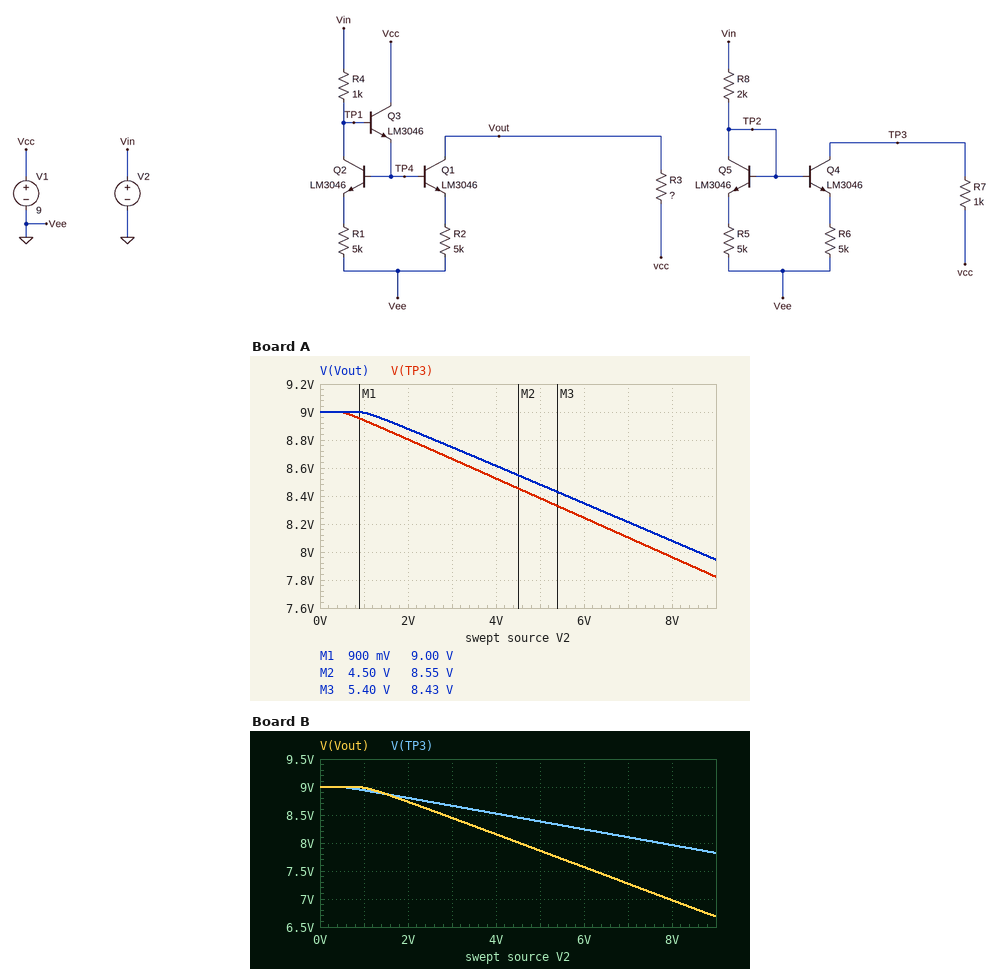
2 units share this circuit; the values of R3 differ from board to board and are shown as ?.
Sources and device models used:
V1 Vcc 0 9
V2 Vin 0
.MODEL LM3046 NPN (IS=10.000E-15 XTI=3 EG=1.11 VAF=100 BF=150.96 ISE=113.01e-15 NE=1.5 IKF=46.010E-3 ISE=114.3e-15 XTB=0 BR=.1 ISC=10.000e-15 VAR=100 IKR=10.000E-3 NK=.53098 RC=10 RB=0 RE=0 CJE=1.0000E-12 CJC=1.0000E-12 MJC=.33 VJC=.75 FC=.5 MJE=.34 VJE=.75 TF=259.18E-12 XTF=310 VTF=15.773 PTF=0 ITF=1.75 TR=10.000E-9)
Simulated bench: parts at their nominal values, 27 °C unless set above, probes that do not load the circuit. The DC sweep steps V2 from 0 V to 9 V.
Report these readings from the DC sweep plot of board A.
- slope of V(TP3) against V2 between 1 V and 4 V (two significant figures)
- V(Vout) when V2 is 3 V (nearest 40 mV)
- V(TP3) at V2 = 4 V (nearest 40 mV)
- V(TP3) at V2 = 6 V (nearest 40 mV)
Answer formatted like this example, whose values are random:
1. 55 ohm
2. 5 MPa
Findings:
1. -0.14 V/V
2. 8.76 V
3. 8.52 V
4. 8.24 V
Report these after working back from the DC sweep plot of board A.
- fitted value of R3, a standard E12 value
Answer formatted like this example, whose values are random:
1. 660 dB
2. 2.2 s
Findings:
1. 820 Ω
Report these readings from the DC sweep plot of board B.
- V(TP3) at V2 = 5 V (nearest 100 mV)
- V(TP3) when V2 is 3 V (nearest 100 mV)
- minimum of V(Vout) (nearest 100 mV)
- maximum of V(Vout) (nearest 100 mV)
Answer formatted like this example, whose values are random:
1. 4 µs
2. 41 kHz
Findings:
1. 8.4 V
2. 8.7 V
3. 6.7 V
4. 9.0 V
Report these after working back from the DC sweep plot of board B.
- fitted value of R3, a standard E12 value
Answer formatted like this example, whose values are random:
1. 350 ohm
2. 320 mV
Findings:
1. 1.8 kΩ
